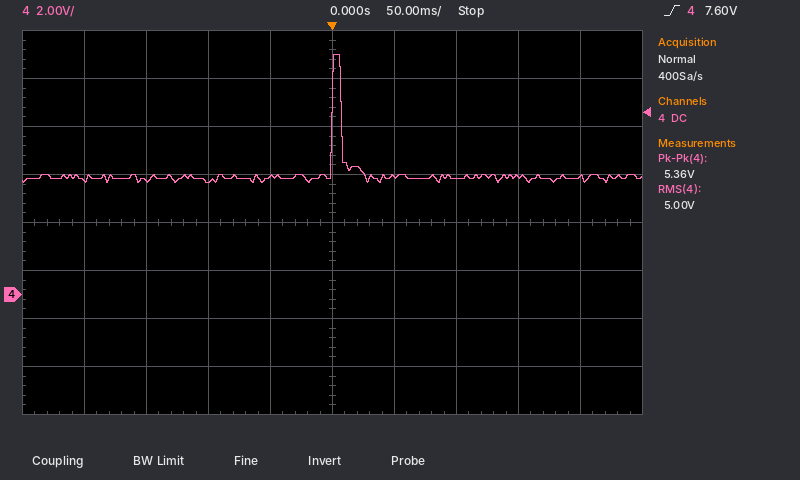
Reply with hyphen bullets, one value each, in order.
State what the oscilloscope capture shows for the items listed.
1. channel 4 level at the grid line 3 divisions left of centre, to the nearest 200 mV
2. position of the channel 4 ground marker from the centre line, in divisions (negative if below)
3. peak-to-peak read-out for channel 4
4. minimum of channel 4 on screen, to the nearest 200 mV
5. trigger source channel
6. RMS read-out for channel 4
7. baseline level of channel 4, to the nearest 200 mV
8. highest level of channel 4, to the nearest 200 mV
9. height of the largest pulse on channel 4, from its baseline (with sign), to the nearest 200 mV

- 4.8 V
- -1.5 div
- 5.36 V
- 4.6 V
- channel 4
- 5.00 V
- 4.8 V
- 10.0 V
- +5.2 V
